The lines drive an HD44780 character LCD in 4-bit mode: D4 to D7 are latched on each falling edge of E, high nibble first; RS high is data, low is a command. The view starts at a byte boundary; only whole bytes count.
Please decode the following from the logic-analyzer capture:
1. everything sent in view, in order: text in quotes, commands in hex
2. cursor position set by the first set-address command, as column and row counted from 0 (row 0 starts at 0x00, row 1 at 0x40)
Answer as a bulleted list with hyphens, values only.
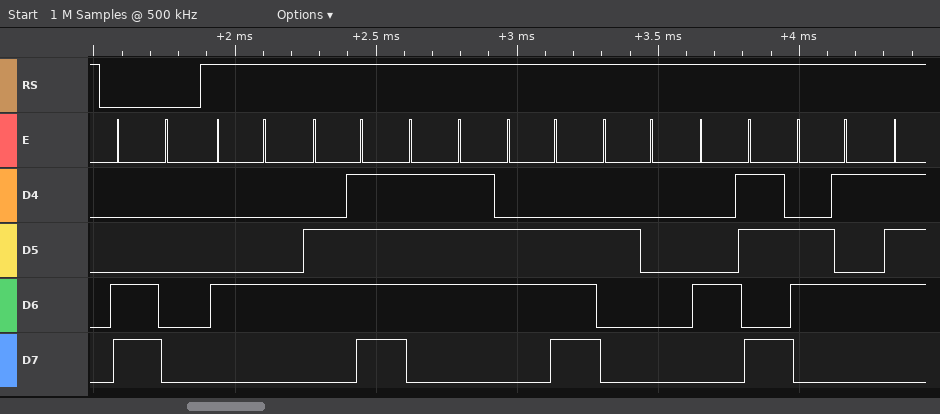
- 0xC0 "Down Ke"
- column 0, row 1
